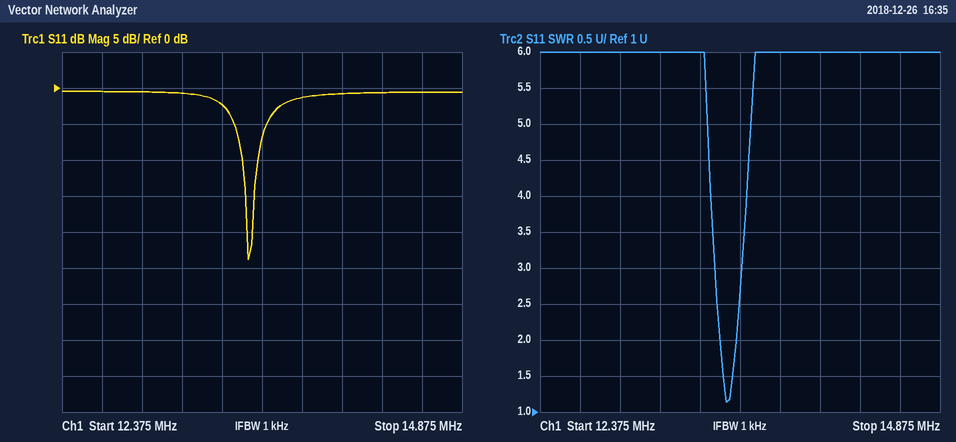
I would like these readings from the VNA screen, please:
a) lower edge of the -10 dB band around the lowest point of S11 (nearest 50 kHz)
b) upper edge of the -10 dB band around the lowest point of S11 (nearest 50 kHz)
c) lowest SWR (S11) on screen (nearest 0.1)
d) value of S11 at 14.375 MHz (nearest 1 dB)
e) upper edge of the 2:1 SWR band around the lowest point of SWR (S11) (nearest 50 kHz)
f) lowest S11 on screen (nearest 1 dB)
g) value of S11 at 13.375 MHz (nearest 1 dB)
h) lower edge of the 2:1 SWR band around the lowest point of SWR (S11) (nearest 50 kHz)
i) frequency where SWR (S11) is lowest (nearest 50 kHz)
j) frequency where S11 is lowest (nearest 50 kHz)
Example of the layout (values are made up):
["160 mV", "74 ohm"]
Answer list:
["13.50 MHz", "13.60 MHz", "1.1", "-1 dB", "13.60 MHz", "-24 dB", "-2 dB", "13.50 MHz", "13.55 MHz", "13.55 MHz"]
